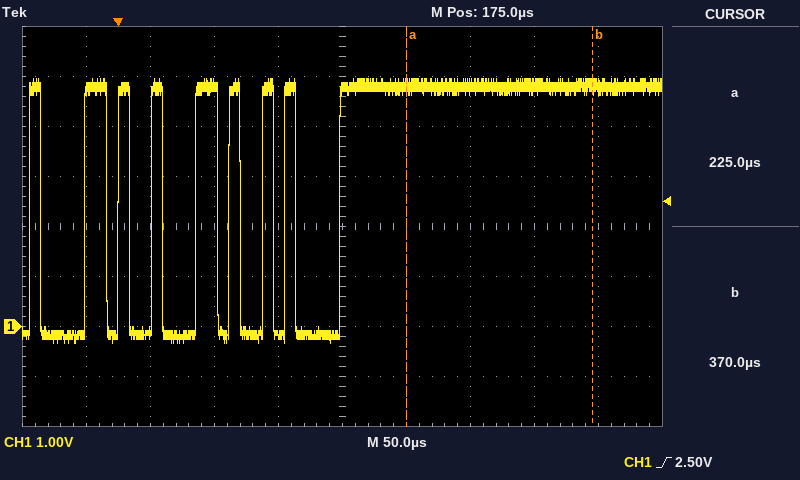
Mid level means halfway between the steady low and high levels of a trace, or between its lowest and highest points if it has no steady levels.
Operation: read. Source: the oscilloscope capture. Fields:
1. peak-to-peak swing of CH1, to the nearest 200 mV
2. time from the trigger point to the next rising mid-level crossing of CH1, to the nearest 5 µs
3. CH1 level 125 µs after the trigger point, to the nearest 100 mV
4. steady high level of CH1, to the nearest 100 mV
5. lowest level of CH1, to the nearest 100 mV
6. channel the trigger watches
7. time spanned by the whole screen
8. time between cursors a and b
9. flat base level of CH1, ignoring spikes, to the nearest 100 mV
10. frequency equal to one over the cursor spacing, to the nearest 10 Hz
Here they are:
5.2 V
25 µs
-200 mV
4.8 V
-300 mV
CH1
500 µs
145 µs
-200 mV
6.90 kHz
